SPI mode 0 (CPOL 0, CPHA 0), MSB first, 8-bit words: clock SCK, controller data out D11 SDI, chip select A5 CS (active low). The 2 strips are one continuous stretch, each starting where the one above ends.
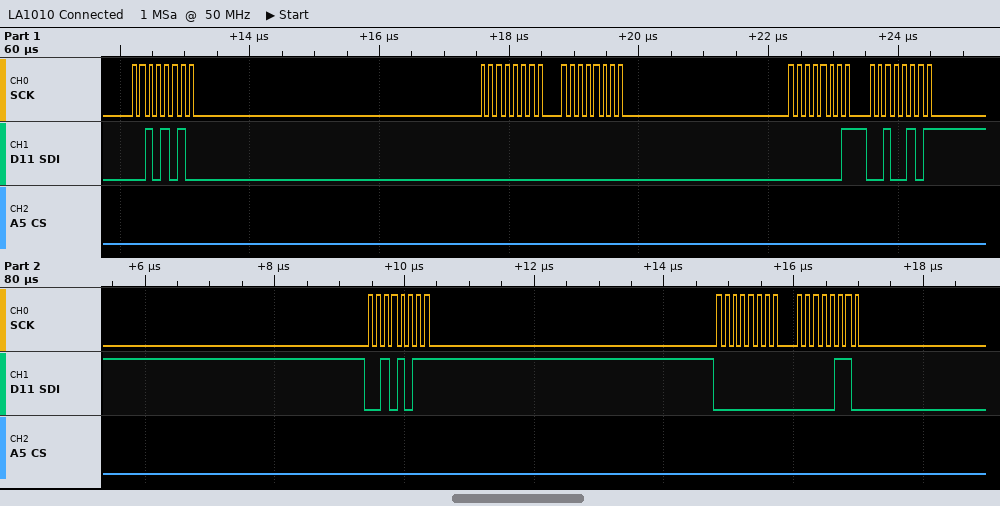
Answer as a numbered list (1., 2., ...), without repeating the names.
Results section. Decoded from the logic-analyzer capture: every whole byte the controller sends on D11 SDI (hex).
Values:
1. 2A 00 00 01 25 2B 00 06
